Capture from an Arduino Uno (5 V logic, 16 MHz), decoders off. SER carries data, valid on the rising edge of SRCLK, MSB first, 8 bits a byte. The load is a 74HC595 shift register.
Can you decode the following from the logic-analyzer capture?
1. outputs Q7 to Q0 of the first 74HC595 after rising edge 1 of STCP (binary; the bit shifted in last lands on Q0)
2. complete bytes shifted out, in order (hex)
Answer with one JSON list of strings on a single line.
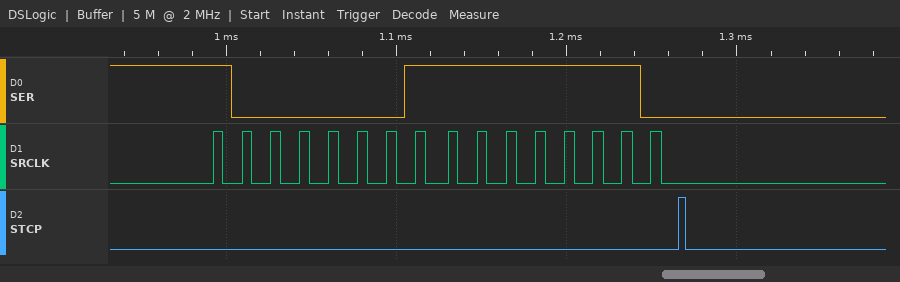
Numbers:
["11111110", "0x81 0xFE"]
